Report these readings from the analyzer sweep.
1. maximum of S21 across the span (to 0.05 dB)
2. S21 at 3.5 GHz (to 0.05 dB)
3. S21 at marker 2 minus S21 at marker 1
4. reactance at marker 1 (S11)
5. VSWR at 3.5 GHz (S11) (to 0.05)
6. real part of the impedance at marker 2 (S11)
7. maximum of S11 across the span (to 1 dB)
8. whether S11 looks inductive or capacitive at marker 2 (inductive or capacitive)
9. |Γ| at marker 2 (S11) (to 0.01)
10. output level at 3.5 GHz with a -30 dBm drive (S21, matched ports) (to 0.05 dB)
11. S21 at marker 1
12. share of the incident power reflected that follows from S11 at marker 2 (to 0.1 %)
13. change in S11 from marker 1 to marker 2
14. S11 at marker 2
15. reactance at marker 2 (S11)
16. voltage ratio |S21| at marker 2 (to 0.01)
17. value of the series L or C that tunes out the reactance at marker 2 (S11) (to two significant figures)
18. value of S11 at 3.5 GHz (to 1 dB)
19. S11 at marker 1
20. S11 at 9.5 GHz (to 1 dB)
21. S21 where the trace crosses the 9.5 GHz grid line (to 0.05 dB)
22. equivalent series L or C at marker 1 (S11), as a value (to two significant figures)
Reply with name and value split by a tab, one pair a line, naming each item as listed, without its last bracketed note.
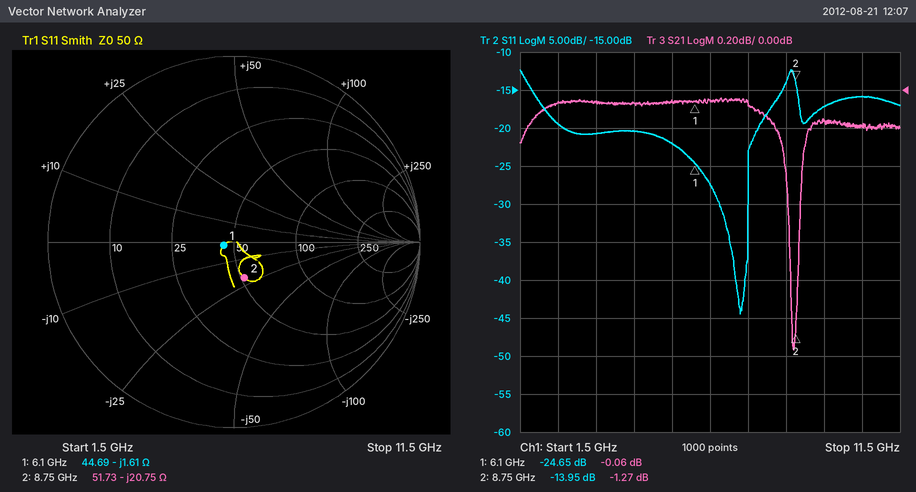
maximum of S21 across the span	-0.05 dB
S21 at 3.5 GHz	-0.05 dB
S21 at marker 2 minus S21 at marker 1	-1.21 dB
reactance at marker 1	-1.61 Ω
VSWR at 3.5 GHz (S11)	1.20
real part of the impedance at marker 2	51.73 Ω
maximum of S11 across the span	-12 dB
whether S11 looks inductive or capacitive at marker 2	capacitive
|Γ| at marker 2 (S11)	0.20
output level at 3.5 GHz with a -30 dBm drive (S21, matched ports)	-30.05 dBm
S21 at marker 1	-0.06 dB
share of the incident power reflected that follows from S11 at marker 2	4.0 %
change in S11 from marker 1 to marker 2	10.70 dB
S11 at marker 2	-13.95 dB
reactance at marker 2	-20.75 Ω
voltage ratio |S21| at marker 2	0.86
value of the series L or C that tunes out the reactance at marker 2 (S11)	380 pH
value of S11 at 3.5 GHz	-21 dB
S11 at marker 1	-24.65 dB
S11 at 9.5 GHz	-17 dB
S21 where the trace crosses the 9.5 GHz grid line	-0.15 dB
equivalent series L or C at marker 1 (S11), as a value	16 pF
